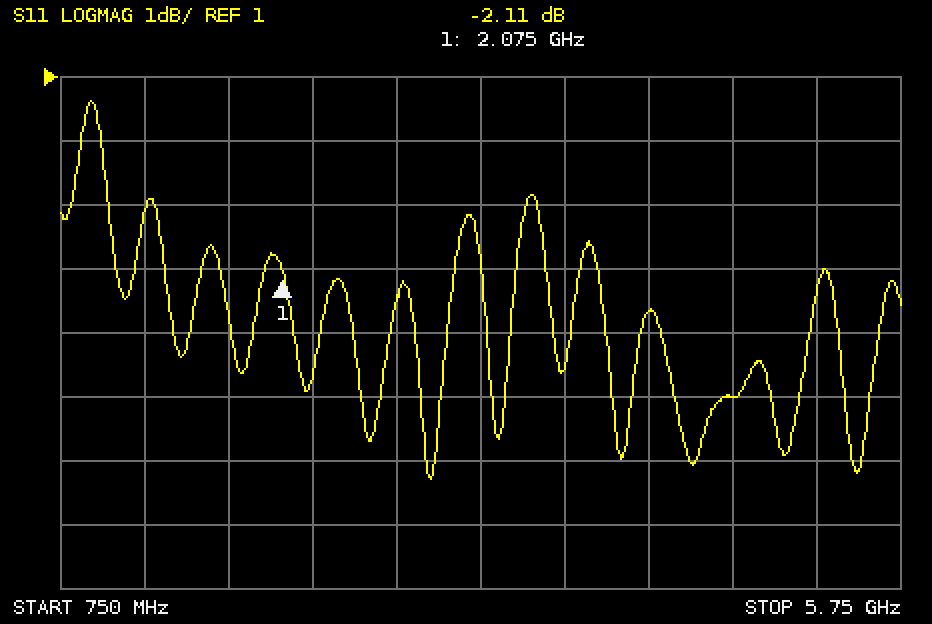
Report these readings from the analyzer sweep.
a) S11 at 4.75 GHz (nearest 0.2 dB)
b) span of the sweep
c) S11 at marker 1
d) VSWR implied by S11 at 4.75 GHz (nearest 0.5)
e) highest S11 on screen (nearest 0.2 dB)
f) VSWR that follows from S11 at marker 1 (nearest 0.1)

-4.0 dB
5 GHz
-2.11 dB
4.5
0.6 dB
8.3
